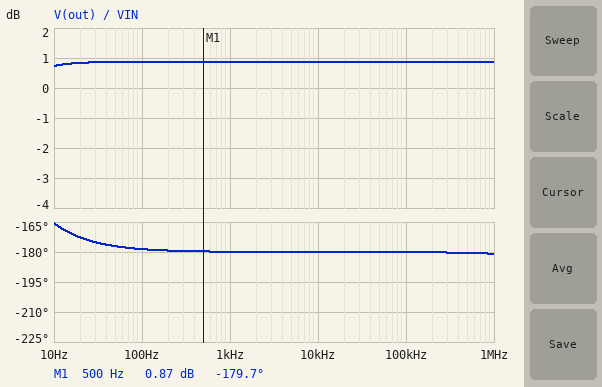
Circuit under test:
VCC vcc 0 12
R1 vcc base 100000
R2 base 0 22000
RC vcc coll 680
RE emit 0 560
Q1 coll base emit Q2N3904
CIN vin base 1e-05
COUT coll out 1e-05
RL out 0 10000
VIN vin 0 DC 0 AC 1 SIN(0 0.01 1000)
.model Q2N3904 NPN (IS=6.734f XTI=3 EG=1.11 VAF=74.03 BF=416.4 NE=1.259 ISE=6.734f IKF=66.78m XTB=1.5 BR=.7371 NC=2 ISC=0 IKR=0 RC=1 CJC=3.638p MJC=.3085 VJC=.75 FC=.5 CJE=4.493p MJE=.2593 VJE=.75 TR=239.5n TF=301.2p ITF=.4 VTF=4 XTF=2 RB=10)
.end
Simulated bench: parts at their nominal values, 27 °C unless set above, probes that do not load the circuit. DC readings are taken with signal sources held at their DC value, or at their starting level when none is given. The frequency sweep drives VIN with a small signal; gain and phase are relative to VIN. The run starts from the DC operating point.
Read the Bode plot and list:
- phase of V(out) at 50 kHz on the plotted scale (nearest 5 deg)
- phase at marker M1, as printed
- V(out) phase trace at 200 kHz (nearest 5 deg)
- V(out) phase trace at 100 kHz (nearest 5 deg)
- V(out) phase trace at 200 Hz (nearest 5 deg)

-180 deg
-179.7 deg
-180 deg
-180 deg
-180 deg
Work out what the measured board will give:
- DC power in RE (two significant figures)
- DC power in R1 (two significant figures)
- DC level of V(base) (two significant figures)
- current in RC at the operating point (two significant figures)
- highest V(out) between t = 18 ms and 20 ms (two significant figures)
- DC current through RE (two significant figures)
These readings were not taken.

2.7 mW
1.0 mW
1.9 V
2.2 mA
11 mV
2.2 mA
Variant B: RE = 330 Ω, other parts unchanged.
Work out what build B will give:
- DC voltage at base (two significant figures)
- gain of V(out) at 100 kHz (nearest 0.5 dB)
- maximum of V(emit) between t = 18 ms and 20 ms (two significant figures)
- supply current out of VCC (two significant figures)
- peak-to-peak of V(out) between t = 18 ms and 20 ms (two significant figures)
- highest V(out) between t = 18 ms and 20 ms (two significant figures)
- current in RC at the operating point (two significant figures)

1.8 V
5.5 dB
1.1 V
3.4 mA
37 mV
19 mV
3.3 mA
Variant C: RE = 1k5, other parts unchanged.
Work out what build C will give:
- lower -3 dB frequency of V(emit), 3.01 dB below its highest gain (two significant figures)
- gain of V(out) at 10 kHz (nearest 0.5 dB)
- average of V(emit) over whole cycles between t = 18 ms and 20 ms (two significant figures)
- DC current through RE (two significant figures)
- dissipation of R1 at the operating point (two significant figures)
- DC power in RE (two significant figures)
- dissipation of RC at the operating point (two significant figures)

950 mHz
-7.5 dB
1.4 V
930 µA
990 µW
1.3 mW
580 µW
